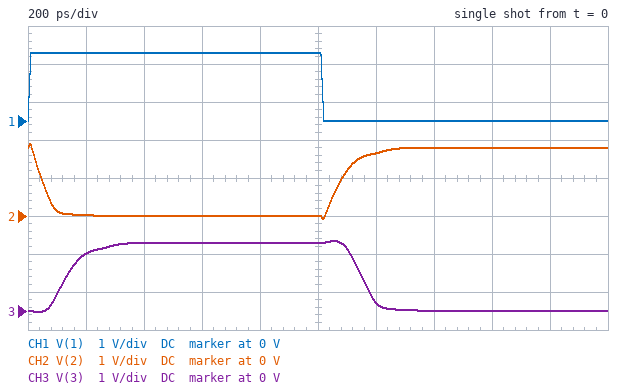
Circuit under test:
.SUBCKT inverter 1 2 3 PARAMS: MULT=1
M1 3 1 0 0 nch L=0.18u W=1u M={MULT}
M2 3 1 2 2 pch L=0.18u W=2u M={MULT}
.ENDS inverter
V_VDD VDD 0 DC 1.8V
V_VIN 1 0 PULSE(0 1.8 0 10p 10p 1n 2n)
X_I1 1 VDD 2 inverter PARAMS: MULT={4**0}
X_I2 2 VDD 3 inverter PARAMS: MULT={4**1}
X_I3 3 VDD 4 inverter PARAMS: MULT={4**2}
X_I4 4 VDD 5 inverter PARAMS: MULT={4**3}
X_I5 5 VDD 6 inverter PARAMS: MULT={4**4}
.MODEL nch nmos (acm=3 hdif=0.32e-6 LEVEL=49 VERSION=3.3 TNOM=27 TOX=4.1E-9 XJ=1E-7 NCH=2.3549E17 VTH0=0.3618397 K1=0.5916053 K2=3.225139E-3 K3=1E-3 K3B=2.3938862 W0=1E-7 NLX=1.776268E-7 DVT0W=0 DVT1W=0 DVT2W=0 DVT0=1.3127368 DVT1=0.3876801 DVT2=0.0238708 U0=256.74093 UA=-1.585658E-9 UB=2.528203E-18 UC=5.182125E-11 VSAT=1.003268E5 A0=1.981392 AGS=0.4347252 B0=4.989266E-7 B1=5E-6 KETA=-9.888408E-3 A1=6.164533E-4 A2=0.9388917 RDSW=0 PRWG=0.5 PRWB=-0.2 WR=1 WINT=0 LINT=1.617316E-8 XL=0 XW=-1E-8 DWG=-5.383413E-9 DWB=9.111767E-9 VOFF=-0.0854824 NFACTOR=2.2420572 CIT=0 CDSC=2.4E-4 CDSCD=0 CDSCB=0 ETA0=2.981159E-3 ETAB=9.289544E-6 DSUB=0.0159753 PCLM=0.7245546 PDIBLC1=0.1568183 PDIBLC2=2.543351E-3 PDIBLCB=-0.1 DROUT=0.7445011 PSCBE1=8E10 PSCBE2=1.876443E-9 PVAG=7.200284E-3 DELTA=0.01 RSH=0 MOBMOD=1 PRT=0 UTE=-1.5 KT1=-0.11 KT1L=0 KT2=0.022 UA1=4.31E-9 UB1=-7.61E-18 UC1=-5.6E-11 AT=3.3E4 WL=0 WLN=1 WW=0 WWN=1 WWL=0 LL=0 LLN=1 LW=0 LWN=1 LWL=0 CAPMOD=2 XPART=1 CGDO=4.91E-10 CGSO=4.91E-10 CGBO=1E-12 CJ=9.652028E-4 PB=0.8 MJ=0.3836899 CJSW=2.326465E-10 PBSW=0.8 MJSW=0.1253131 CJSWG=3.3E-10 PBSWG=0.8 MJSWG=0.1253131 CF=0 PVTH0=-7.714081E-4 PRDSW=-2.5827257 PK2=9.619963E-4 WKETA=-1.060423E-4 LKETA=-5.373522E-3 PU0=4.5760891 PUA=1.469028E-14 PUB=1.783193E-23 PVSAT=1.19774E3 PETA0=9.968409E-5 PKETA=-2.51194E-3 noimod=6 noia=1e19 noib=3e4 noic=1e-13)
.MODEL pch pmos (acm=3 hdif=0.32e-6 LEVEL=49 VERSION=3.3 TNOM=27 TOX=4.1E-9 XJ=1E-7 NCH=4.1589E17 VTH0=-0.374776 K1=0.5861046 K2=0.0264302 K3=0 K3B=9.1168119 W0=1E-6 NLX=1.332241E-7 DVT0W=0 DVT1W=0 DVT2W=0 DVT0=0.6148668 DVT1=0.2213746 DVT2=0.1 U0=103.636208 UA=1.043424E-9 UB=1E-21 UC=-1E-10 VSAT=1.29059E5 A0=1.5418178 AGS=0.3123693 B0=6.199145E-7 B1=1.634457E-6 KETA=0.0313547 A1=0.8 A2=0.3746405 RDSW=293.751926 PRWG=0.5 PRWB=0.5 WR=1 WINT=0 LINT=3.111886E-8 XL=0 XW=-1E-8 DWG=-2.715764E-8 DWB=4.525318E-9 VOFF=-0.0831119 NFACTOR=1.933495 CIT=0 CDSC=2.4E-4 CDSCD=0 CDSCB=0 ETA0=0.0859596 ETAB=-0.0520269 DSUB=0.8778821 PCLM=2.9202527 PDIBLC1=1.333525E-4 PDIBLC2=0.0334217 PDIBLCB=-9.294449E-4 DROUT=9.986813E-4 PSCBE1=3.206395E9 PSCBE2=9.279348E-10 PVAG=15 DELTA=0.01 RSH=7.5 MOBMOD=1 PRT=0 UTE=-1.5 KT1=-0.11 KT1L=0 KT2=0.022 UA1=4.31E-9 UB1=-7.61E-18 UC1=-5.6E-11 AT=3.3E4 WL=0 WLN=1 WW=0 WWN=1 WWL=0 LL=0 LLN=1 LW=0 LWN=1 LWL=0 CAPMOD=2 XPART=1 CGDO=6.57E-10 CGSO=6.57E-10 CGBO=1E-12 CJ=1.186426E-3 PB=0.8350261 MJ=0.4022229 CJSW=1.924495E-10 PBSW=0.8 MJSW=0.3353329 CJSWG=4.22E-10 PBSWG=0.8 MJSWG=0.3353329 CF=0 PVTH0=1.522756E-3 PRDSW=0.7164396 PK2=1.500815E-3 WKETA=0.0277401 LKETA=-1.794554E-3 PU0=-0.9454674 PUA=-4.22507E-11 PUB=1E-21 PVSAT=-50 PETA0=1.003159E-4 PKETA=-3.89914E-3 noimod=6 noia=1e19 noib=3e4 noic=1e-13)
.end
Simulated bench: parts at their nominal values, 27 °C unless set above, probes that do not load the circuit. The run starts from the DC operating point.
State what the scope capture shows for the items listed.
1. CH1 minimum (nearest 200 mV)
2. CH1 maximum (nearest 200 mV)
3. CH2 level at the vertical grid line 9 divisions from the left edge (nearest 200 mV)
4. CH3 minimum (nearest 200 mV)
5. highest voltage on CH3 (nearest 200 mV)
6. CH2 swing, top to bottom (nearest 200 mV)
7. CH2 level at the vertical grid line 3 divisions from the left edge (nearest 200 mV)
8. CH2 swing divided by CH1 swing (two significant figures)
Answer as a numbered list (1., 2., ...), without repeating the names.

1. 0 V
2. 1.8 V
3. 1.8 V
4. 0 V
5. 1.8 V
6. 2.0 V
7. 0 V
8. 1.1
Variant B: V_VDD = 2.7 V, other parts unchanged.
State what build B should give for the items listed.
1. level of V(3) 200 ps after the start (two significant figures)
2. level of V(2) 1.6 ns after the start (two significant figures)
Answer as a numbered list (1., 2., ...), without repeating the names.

1. 2.2 V
2. 2.7 V
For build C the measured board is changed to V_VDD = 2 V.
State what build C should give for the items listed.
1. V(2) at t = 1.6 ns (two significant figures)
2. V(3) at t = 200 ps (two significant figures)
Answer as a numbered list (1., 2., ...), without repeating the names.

1. 2.0 V
2. 1.7 V
